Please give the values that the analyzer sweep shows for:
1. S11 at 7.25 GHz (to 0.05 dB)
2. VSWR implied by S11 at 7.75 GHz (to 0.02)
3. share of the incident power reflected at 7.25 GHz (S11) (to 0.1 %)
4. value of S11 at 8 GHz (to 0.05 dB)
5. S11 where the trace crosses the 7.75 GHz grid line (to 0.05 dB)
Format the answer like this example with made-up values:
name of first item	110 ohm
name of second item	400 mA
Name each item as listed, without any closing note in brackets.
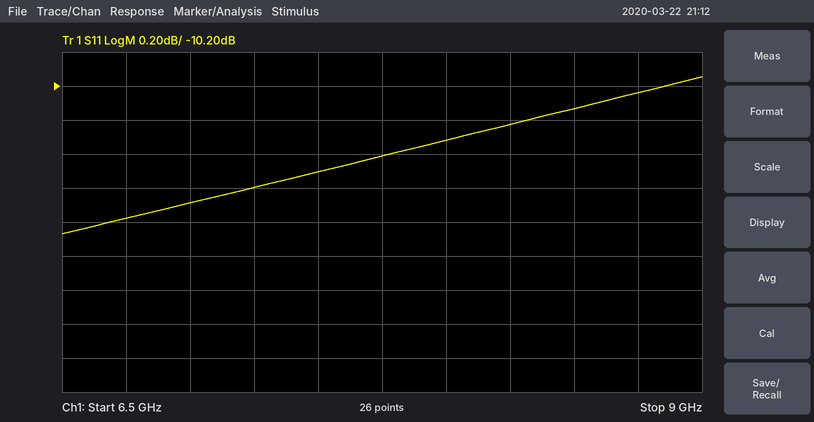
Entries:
S11 at 7.25 GHz	-10.80 dB
VSWR implied by S11 at 7.75 GHz	1.84
share of the incident power reflected at 7.25 GHz (S11)	8.3 %
value of S11 at 8 GHz	-10.50 dB
S11 where the trace crosses the 7.75 GHz grid line	-10.60 dB
